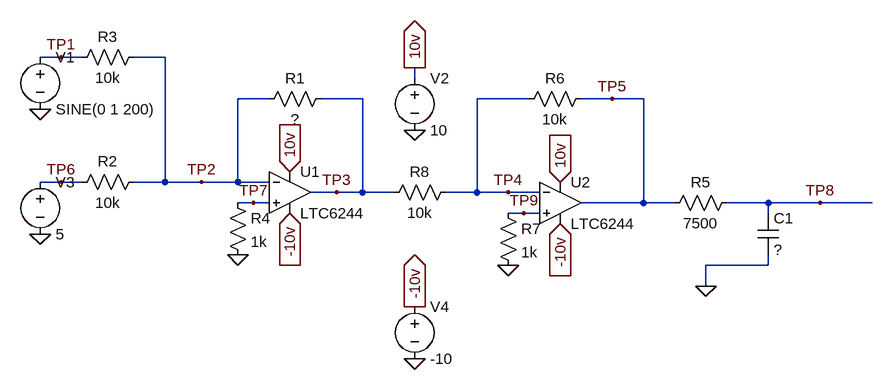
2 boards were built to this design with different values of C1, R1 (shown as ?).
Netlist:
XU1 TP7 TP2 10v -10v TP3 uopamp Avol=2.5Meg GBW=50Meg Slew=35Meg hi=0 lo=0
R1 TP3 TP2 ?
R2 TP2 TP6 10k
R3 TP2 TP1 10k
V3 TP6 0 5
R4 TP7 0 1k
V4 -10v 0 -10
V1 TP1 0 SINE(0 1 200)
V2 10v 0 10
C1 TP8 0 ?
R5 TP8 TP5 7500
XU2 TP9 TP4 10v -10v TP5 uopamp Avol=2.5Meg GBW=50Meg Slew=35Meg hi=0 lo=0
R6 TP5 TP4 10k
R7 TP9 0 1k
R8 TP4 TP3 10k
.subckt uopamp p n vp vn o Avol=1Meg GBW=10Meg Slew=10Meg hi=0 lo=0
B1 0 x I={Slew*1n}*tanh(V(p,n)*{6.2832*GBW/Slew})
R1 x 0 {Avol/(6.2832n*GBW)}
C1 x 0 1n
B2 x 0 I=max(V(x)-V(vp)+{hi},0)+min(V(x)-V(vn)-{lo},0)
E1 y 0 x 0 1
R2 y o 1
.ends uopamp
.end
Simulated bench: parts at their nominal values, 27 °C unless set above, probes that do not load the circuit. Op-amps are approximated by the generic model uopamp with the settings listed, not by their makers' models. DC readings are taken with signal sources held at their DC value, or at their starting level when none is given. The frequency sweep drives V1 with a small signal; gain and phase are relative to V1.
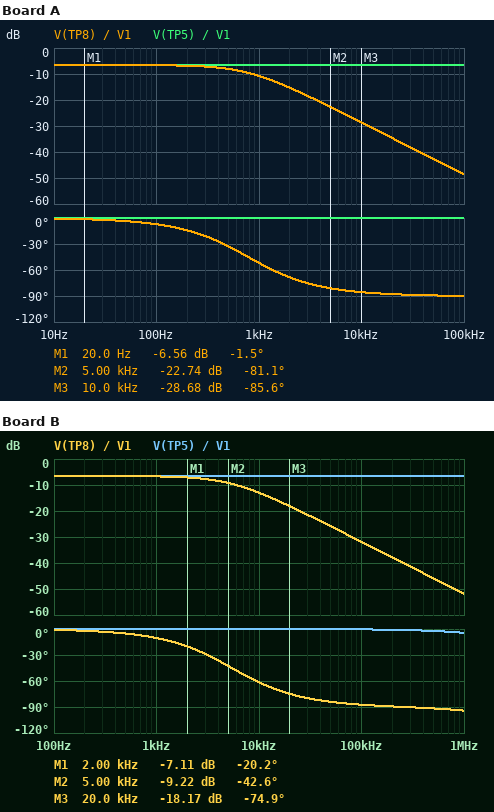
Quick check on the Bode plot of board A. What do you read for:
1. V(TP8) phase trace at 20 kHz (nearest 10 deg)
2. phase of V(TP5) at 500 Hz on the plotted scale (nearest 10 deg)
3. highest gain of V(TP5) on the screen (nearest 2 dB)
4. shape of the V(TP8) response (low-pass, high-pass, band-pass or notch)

-90 deg
0 deg
-6 dB
low-pass
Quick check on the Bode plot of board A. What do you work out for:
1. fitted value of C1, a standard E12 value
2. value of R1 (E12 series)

27 nF
4.7 kΩ
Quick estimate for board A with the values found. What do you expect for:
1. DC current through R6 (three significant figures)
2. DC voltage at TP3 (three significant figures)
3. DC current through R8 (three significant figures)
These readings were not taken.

235 µA
-2.35 V
235 µA
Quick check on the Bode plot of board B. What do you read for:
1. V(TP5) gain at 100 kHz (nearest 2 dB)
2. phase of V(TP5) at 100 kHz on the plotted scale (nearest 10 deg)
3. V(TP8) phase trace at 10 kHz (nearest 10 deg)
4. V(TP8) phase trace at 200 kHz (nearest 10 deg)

-6 dB
0 deg
-60 deg
-90 deg
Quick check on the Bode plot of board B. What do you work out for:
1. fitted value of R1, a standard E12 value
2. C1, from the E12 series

4.7 kΩ
3.9 nF
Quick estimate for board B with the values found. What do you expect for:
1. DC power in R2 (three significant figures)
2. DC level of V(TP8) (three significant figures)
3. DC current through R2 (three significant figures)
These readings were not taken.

2.50 mW
2.35 V
500 µA
